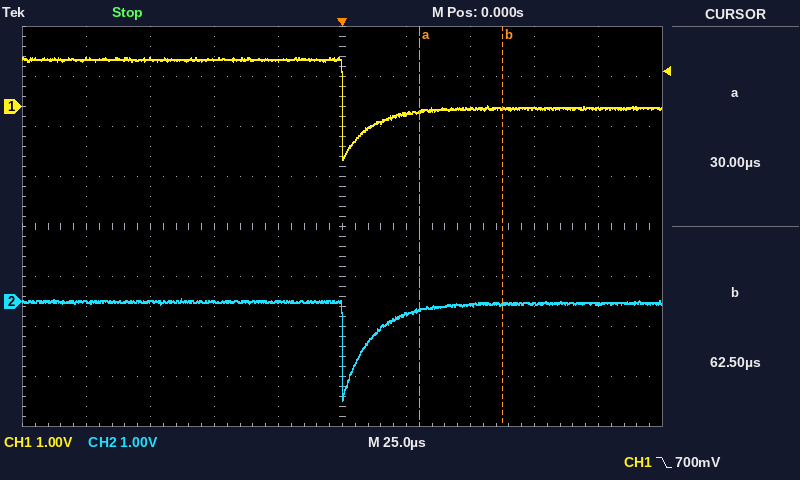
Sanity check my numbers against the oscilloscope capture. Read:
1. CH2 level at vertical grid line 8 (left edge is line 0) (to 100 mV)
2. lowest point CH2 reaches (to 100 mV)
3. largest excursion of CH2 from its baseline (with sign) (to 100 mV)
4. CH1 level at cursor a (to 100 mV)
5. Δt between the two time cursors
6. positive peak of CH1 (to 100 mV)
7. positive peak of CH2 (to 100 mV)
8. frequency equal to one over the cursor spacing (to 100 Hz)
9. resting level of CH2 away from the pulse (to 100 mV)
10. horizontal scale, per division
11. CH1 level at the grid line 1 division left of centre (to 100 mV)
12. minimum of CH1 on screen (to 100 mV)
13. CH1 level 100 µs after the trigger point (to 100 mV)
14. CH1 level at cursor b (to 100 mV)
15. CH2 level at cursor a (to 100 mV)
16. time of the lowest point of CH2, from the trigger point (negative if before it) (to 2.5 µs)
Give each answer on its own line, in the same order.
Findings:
0.0 V
-2.0 V
-2.0 V
-100 mV
32.5 µs
1.0 V
100 mV
30.8 kHz
0.0 V
25 µs
900 mV
-1.1 V
0.0 V
0.0 V
-200 mV
0.0 µs
